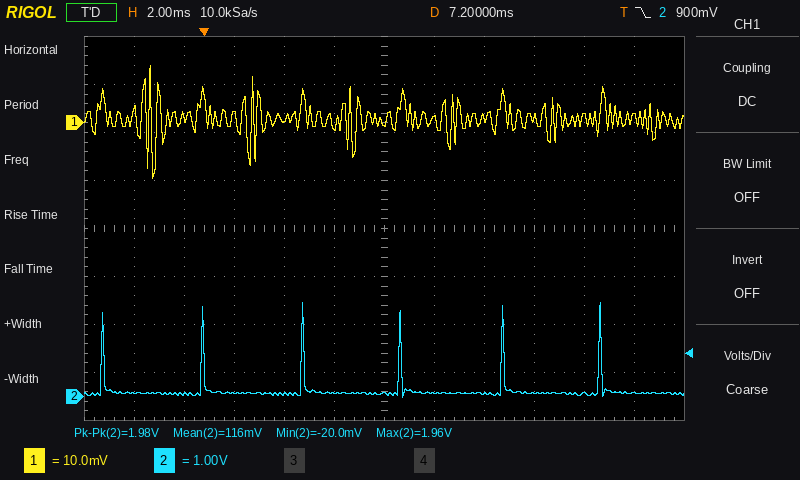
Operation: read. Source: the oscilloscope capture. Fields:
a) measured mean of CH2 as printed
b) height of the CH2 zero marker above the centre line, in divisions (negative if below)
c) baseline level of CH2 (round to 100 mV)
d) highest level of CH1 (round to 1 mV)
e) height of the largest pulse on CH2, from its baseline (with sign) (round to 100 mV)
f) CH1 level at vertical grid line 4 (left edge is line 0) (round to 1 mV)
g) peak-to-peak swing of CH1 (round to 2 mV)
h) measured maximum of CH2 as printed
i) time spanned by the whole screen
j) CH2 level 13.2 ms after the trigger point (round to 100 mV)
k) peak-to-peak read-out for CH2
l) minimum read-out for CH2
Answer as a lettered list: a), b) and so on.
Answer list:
a) 116 mV
b) -3.5 div
c) 100 mV
d) 12 mV
e) +1.9 V
f) 1 mV
g) 24 mV
h) 1.96 V
i) 24 ms
j) 100 mV
k) 1.98 V
l) -20.0 mV
